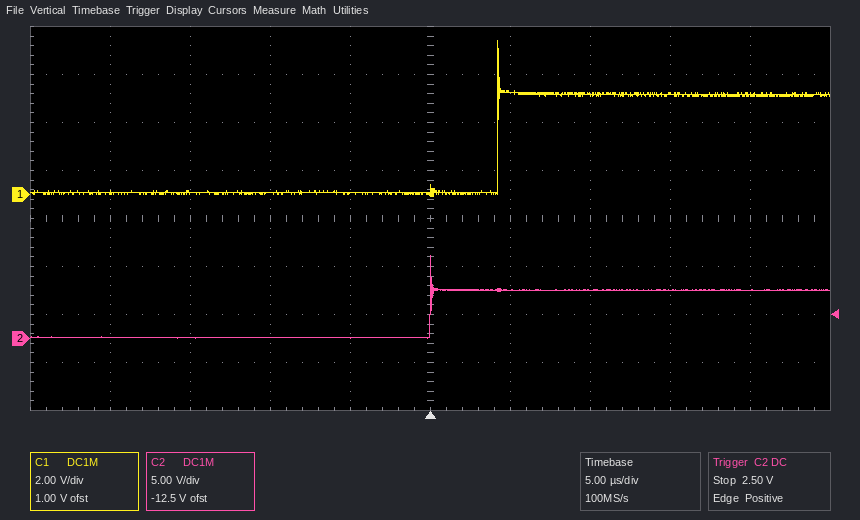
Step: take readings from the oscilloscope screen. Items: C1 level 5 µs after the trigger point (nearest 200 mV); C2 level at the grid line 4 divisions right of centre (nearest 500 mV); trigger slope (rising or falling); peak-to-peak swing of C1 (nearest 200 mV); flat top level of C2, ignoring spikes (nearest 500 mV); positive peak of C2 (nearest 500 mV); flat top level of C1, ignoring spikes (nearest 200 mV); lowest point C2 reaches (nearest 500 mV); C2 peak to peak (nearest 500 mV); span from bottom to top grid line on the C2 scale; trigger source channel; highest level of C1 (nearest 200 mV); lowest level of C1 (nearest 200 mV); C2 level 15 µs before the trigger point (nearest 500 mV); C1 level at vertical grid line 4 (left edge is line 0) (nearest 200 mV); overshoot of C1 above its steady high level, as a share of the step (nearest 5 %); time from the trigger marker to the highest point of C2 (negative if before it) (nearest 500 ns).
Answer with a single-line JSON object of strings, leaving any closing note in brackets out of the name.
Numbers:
{"C1 level 5 µs after the trigger point": "4.2 V", "C2 level at the grid line 4 divisions right of centre": "5.0 V", "trigger slope": "rising", "peak-to-peak swing of C1": "6.4 V", "flat top level of C2, ignoring spikes": "5.0 V", "positive peak of C2": "8.5 V", "flat top level of C1, ignoring spikes": "4.2 V", "lowest point C2 reaches": "0.0 V", "C2 peak to peak": "8.5 V", "span from bottom to top grid line on the C2 scale": "40 V", "trigger source channel": "C2", "highest level of C1": "6.4 V", "lowest level of C1": "0.0 V", "C2 level 15 µs before the trigger point": "0.0 V", "C1 level at vertical grid line 4 (left edge is line 0)": "0.0 V", "overshoot of C1 above its steady high level, as a share of the step": "55 %", "time from the trigger marker to the highest point of C2 (negative if before it)": "0.0 µs"}
